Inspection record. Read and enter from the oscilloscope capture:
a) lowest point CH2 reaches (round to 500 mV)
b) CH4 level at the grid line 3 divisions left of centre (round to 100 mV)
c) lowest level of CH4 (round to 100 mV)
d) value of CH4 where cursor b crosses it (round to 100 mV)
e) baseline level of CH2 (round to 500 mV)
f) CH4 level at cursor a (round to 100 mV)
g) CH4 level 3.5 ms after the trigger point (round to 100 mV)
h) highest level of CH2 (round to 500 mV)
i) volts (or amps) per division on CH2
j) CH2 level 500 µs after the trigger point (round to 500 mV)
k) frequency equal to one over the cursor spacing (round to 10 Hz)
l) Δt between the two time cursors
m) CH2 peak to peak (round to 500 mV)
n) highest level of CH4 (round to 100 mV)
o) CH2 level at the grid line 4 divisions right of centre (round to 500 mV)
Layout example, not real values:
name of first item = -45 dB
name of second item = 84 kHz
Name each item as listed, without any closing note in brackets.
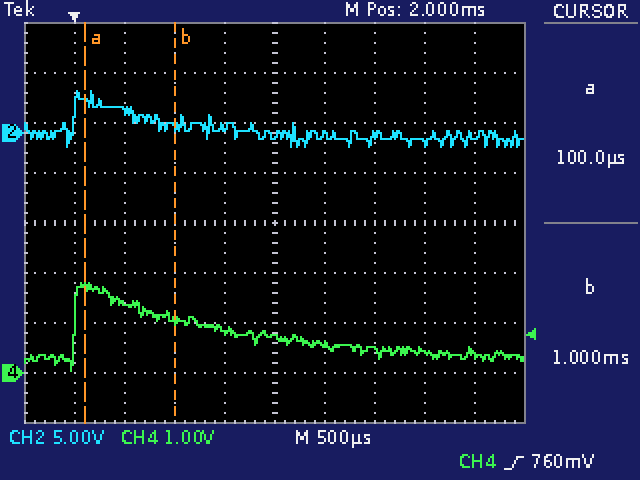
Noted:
lowest point CH2 reaches = -1.5 V
CH4 level at the grid line 3 divisions left of centre = 1.4 V
lowest level of CH4 = 0.0 V
value of CH4 where cursor b crosses it = 1.1 V
baseline level of CH2 = 0.0 V
CH4 level at cursor a = 1.7 V
CH4 level 3.5 ms after the trigger point = 400 mV
highest level of CH2 = 4.0 V
volts (or amps) per division on CH2 = 5 V
CH2 level 500 µs after the trigger point = 2.0 V
frequency equal to one over the cursor spacing = 1.11 kHz
Δt between the two time cursors = 900 µs
CH2 peak to peak = 5.5 V
highest level of CH4 = 1.8 V
CH2 level at the grid line 4 divisions right of centre = -500 mV
